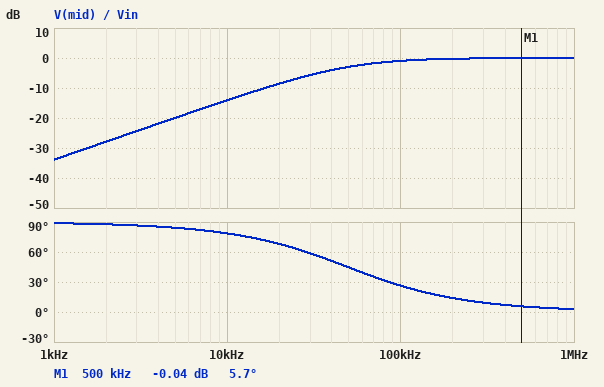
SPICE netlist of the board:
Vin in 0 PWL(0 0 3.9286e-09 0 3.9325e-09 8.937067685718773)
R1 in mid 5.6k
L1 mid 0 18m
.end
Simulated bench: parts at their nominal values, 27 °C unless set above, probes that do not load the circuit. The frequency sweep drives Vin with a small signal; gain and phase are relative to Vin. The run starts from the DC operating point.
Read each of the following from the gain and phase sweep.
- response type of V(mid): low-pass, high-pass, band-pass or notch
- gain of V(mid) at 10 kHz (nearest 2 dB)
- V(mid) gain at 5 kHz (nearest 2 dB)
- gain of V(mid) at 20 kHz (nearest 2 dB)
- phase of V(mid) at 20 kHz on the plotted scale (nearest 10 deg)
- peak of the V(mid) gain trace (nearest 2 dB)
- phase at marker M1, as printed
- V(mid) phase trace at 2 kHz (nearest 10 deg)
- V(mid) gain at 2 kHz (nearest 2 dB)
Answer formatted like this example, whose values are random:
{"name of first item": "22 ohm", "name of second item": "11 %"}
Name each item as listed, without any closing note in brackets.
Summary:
{"response type of V(mid): low-pass, high-pass, band-pass or notch": "high-pass", "gain of V(mid) at 10 kHz": "-14 dB", "V(mid) gain at 5 kHz": "-20 dB", "gain of V(mid) at 20 kHz": "-8 dB", "phase of V(mid) at 20 kHz on the plotted scale": "70 deg", "peak of the V(mid) gain trace": "0 dB", "phase at marker M1, as printed": "5.7 deg", "V(mid) phase trace at 2 kHz": "90 deg", "V(mid) gain at 2 kHz": "-28 dB"}
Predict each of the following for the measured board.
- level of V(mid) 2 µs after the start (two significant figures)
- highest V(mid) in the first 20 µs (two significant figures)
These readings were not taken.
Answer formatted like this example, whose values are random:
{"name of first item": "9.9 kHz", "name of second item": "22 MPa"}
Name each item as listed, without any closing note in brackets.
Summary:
{"level of V(mid) 2 µs after the start": "4.8 V", "highest V(mid) in the first 20 µs": "8.9 V"}
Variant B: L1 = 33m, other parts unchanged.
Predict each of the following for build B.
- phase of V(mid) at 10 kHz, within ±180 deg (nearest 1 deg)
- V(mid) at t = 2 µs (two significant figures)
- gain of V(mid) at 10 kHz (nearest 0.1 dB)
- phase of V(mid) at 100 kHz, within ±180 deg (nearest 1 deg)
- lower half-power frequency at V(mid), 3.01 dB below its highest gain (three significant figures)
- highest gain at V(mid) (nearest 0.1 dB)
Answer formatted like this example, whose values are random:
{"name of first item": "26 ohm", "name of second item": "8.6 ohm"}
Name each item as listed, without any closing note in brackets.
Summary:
{"phase of V(mid) at 10 kHz, within ±180 deg": "70 deg", "V(mid) at t = 2 µs": "6.4 V", "gain of V(mid) at 10 kHz": "-9.2 dB", "phase of V(mid) at 100 kHz, within ±180 deg": "15 deg", "lower half-power frequency at V(mid), 3.01 dB below its highest gain": "27.0 kHz", "highest gain at V(mid)": "0 dB"}
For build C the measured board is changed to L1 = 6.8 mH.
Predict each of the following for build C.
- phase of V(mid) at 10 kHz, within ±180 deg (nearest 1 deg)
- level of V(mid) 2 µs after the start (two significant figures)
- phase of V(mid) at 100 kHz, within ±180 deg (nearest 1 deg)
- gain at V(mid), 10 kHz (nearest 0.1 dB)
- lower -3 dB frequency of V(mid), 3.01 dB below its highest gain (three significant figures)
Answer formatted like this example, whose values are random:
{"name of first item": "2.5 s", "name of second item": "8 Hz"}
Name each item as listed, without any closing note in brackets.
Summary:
{"phase of V(mid) at 10 kHz, within ±180 deg": "86 deg", "level of V(mid) 2 µs after the start": "1.7 V", "phase of V(mid) at 100 kHz, within ±180 deg": "53 deg", "gain at V(mid), 10 kHz": "-22.4 dB", "lower -3 dB frequency of V(mid), 3.01 dB below its highest gain": "131 kHz"}
